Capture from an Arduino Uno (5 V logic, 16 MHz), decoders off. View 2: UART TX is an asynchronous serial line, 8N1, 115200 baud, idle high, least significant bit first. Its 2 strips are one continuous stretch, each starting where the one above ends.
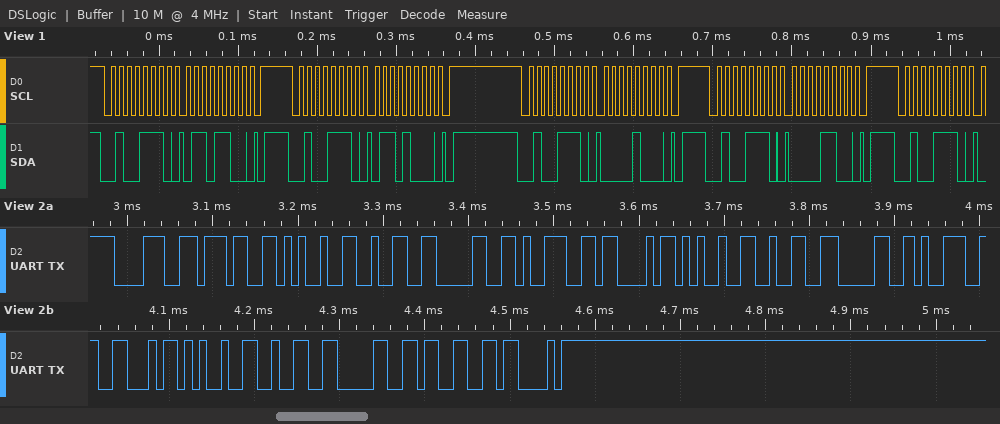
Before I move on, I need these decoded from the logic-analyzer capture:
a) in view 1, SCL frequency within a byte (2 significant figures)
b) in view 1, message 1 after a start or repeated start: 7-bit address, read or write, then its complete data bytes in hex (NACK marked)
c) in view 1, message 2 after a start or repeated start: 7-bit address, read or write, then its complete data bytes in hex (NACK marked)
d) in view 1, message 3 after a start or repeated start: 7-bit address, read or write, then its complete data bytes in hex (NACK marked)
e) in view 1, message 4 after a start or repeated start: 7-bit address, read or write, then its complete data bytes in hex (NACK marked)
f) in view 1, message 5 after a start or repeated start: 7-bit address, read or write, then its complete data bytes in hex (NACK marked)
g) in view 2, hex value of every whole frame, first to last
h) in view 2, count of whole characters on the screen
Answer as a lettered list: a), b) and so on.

a) 100 kHz
b) 0x27 write: 6C
c) 0x27 write: 68
d) 0x27 write: 08
e) 0x27 write: 0C
f) 0x27 write
g) 0x38 0x37 0x25 0x32 0x30 0x39 0x43 0x25 0x32 0x30 0x39 0x46 0x25 0x32 0x30 0x33 0x43
h) 17
